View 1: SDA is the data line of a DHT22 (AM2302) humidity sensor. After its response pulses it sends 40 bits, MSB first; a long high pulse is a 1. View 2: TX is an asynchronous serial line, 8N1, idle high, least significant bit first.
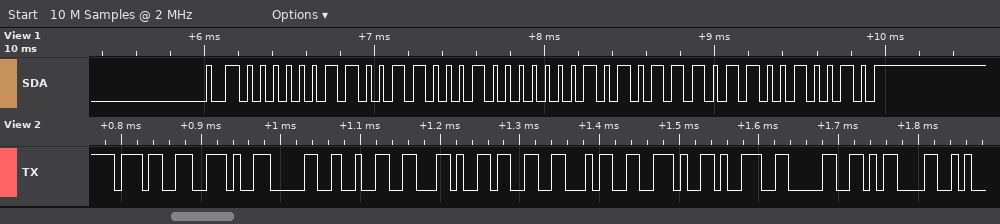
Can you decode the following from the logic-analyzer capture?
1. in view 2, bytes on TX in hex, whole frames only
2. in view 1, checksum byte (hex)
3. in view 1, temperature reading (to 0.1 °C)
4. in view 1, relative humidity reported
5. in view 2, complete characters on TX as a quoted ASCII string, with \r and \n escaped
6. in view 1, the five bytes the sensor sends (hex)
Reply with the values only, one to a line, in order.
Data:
37 2E 30 32 2C 33 34 2E 39 30 0D
0x92
34.9 °C
81.7 %
"7.02,34.90\r"
03 31 01 5D 92
